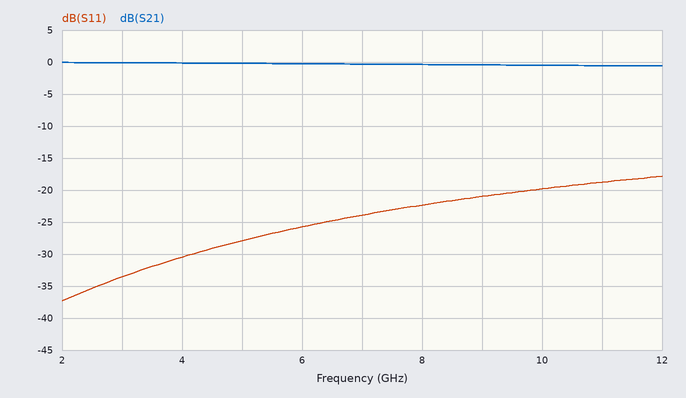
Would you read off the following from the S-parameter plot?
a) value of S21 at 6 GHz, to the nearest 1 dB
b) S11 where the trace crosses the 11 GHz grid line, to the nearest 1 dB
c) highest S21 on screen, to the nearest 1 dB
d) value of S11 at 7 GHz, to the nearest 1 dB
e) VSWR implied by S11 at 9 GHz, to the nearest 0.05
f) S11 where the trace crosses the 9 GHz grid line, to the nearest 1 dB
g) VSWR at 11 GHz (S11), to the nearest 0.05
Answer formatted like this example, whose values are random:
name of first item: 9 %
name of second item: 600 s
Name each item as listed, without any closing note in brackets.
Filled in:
value of S21 at 6 GHz, to the nearest 1 dB: 0 dB
S11 where the trace crosses the 11 GHz grid line, to the nearest 1 dB: -19 dB
highest S21 on screen, to the nearest 1 dB: 0 dB
value of S11 at 7 GHz, to the nearest 1 dB: -24 dB
VSWR implied by S11 at 9 GHz, to the nearest 0.05: 1.20
S11 where the trace crosses the 9 GHz grid line, to the nearest 1 dB: -21 dB
VSWR at 11 GHz (S11), to the nearest 0.05: 1.25
